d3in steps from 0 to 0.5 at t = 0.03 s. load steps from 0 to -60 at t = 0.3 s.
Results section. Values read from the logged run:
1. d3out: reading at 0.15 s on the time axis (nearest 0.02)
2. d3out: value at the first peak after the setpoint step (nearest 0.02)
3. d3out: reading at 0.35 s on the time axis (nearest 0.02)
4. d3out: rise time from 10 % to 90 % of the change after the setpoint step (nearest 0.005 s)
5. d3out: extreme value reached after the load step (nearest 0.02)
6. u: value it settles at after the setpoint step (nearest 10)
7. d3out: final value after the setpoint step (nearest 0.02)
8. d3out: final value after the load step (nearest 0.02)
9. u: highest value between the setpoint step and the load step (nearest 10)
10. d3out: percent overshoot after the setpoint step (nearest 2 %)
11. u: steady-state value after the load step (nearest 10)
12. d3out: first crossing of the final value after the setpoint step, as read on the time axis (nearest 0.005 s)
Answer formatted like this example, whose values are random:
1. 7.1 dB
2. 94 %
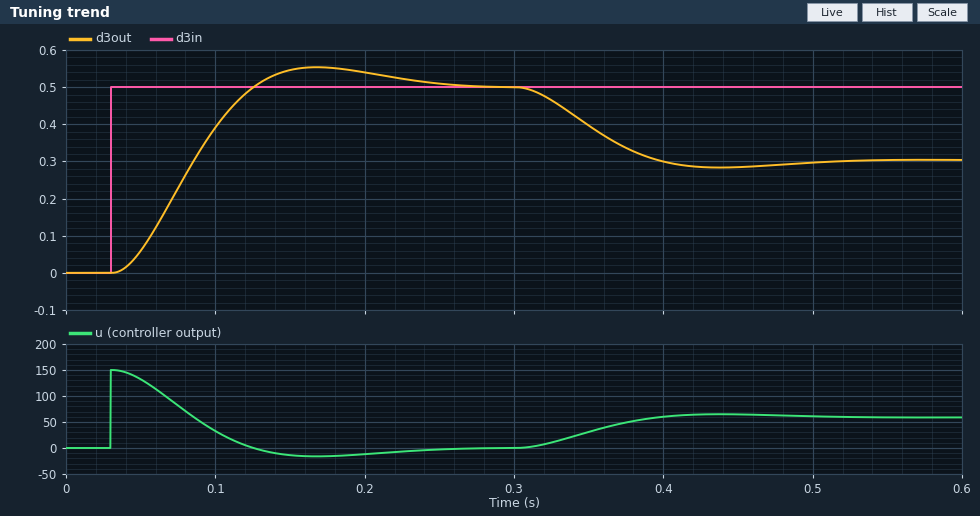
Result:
1. 0.54
2. 0.56
3. 0.40
4. 0.065 s
5. 0.28
6. 0
7. 0.50
8. 0.30
9. 150
10. 10 %
11. 60
12. 0.125 s
